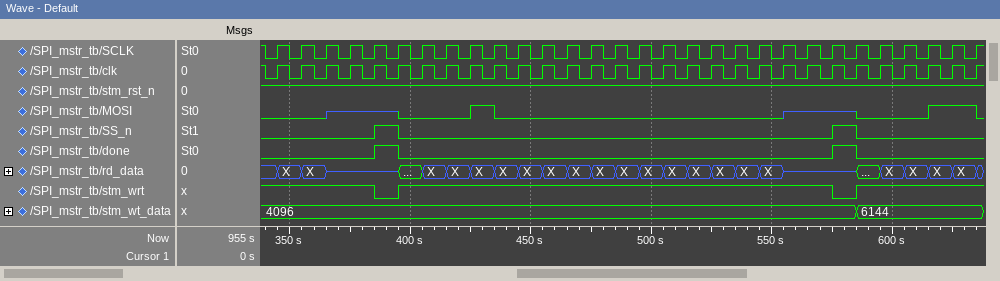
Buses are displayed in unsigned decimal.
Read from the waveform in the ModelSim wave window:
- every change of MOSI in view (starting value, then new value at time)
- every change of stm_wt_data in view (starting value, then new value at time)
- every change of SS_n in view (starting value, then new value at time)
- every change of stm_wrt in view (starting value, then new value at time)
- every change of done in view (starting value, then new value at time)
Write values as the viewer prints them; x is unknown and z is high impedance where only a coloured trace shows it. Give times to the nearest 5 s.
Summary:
0, z at 365 s, 0 at 395 s, 1 at 425 s, 0 at 435 s, z at 555 s, 0 at 585 s, 1 at 615 s, 0 at 635 s
4096, 6144 at 585 s
0, 1 at 385 s, 0 at 395 s, 1 at 575 s, 0 at 585 s
1, 0 at 385 s, 1 at 395 s, 0 at 575 s, 1 at 585 s
0, 1 at 385 s, 0 at 395 s, 1 at 575 s, 0 at 585 s
